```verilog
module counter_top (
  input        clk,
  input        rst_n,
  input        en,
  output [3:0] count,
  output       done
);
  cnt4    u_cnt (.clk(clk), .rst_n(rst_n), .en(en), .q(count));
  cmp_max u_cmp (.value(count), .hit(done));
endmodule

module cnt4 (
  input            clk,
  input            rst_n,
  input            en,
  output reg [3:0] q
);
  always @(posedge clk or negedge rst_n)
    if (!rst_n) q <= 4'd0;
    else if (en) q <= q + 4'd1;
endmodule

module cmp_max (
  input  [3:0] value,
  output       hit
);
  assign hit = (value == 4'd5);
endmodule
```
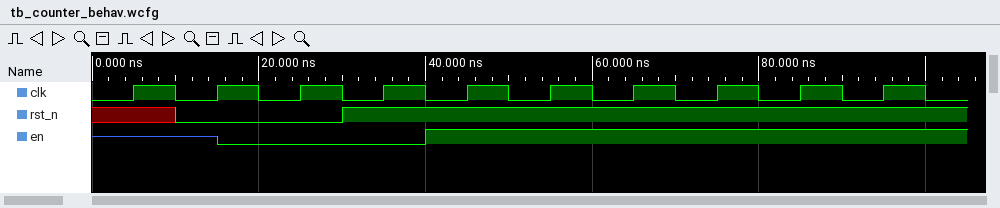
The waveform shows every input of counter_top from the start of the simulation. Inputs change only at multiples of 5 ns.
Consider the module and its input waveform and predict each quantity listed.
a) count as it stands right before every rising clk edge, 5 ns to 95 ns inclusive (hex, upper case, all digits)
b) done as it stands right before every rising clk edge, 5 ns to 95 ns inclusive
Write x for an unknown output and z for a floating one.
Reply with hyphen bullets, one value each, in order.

- x, 0, 0, 0, 0, 1, 2, 3, 4, 5
- x 0 0 0 0 0 0 0 0 1
